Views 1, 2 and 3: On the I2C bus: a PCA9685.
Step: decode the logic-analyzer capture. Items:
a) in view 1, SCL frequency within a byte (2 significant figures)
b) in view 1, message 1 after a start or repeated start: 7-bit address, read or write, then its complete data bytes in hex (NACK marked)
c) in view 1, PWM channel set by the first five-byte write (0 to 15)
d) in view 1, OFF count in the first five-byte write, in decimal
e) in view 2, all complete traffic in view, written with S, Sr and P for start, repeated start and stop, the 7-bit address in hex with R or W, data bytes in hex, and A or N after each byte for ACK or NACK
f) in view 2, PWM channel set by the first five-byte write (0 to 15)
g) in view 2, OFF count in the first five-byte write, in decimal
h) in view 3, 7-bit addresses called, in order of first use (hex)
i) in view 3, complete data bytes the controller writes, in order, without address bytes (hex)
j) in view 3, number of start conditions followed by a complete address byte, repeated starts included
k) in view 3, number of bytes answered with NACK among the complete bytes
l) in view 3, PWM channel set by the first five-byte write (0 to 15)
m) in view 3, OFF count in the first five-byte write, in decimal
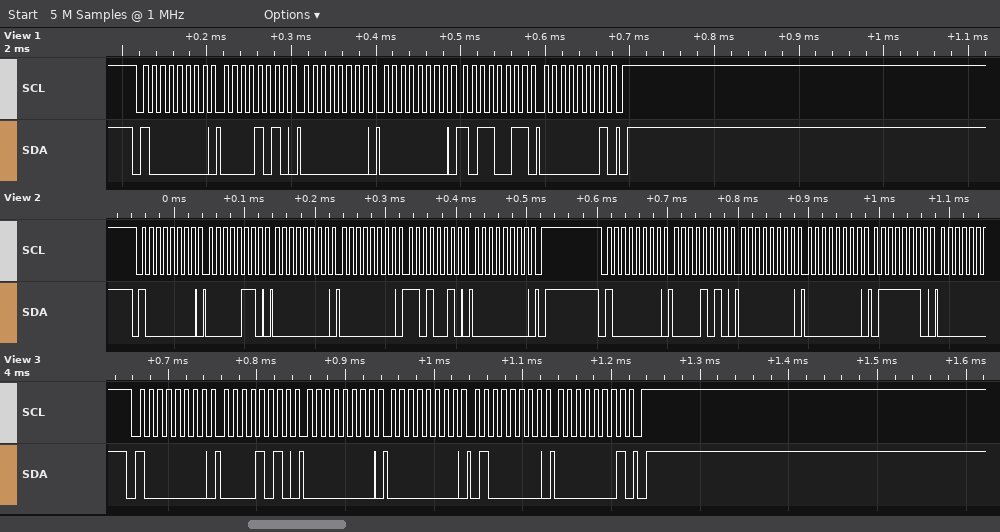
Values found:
100 kHz
0x40 write: 0A 00 00 B3 01
1
435
S 40W A 06 A 00 A 00 A D2 A 00 A P S 40W A 0A A 00 A 00 A 7E A
0
210
0x40
0A 00 00 40 01
1
0
1
320
